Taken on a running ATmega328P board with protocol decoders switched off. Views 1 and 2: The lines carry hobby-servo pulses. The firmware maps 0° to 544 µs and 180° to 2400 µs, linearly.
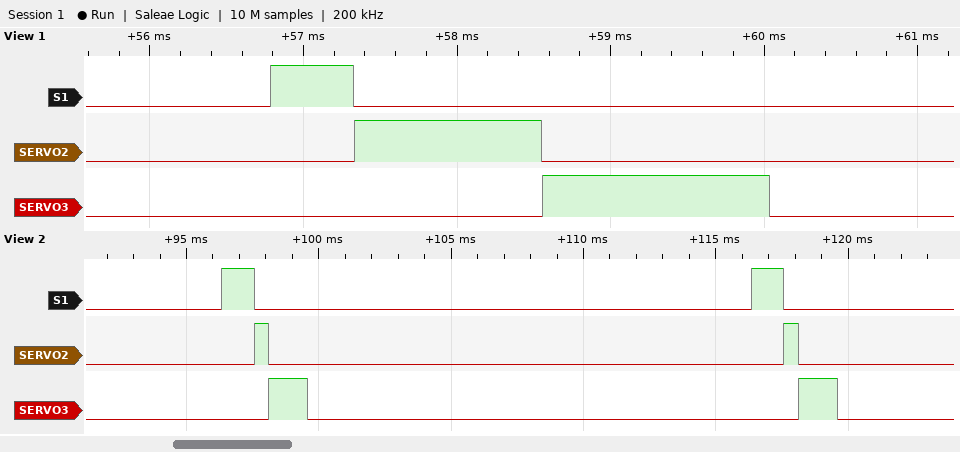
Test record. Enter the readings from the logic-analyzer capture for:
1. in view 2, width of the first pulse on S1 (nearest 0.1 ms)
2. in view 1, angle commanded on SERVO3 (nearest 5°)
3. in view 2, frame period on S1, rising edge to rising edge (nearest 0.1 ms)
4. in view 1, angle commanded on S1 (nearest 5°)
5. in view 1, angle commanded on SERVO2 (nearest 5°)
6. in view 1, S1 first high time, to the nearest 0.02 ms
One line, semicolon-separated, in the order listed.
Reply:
1.2 ms; 90°; 20.0 ms; 0°; 65°; 0.54 ms
